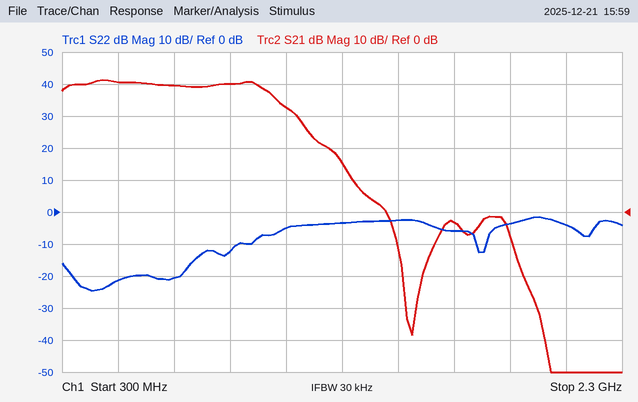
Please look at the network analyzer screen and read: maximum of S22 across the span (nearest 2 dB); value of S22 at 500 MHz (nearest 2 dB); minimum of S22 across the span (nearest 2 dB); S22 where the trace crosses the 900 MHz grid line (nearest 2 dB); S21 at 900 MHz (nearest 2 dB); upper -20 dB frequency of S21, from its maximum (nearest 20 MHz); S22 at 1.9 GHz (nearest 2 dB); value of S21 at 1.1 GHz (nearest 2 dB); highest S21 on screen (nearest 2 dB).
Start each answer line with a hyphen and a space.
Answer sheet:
- -2 dB
- -22 dB
- -24 dB
- -12 dB
- 40 dB
- 1.22 GHz
- -4 dB
- 32 dB
- 42 dB
